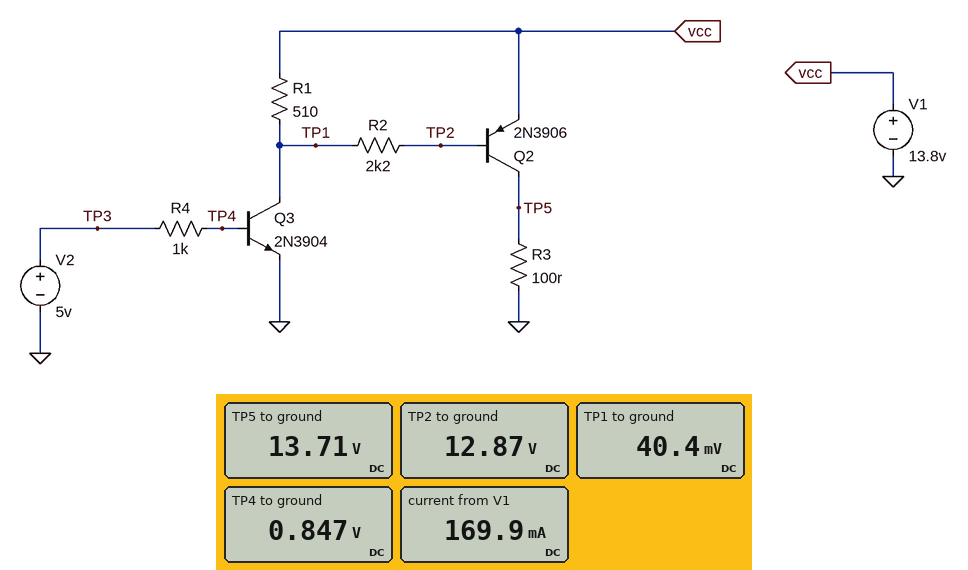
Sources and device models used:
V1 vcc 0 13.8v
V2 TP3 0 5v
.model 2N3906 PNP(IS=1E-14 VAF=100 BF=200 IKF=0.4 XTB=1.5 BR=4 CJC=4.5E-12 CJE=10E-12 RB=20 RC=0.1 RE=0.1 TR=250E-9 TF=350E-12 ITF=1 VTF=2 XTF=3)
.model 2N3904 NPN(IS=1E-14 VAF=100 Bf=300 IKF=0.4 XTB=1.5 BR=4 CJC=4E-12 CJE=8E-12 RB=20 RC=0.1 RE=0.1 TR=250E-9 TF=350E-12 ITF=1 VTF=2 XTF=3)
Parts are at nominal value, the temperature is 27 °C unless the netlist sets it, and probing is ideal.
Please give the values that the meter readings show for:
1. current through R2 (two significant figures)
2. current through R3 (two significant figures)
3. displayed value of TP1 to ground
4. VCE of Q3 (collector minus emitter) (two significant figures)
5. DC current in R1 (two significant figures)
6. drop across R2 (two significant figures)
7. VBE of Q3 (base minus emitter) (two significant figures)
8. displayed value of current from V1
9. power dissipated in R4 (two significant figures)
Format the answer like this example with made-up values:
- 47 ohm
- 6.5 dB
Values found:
- 5.8 mA
- 140 mA
- 40.4 mV
- 40 mV
- 27 mA
- 13 V
- 850 mV
- 169.9 mA
- 17 mW
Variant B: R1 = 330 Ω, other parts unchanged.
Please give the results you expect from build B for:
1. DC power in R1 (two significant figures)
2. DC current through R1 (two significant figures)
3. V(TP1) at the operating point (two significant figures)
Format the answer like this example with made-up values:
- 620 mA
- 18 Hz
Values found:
- 570 mW
- 42 mA
- 51 mV
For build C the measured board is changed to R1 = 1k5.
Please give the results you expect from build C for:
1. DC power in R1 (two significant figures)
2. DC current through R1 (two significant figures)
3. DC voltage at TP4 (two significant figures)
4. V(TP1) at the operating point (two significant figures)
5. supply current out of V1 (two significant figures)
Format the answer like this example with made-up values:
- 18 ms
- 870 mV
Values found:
- 130 mW
- 9.2 mA
- 830 mV
- 25 mV
- 150 mA
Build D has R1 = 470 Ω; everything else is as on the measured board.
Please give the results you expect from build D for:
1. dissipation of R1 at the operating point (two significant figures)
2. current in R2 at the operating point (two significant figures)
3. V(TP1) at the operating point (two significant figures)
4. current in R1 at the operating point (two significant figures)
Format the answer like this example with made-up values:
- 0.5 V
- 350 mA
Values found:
- 400 mW
- 5.8 mA
- 42 mV
- 29 mA
